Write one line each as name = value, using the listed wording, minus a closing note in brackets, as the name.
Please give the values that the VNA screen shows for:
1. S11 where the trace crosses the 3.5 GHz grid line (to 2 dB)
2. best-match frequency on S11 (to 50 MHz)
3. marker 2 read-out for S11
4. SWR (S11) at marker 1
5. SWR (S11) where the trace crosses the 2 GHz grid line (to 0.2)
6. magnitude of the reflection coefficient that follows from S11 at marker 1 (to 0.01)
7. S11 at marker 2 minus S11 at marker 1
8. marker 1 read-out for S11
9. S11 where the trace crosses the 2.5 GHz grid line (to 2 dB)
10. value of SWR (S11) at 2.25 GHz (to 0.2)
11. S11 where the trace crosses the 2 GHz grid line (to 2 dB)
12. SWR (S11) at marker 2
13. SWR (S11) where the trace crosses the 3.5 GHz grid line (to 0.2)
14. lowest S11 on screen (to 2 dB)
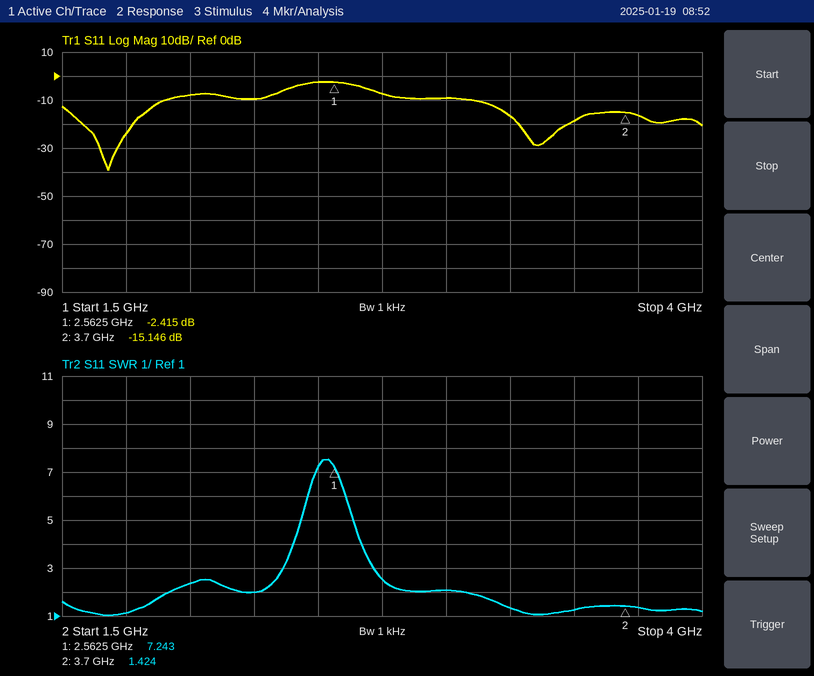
S11 where the trace crosses the 3.5 GHz grid line = -18 dB
best-match frequency on S11 = 1.70 GHz
marker 2 read-out for S11 = -15.146 dB
SWR (S11) at marker 1 = 7.243
SWR (S11) where the trace crosses the 2 GHz grid line = 2.4
magnitude of the reflection coefficient that follows from S11 at marker 1 = 0.76
S11 at marker 2 minus S11 at marker 1 = -12.731 dB
marker 1 read-out for S11 = -2.415 dB
S11 where the trace crosses the 2.5 GHz grid line = -2 dB
value of SWR (S11) at 2.25 GHz = 2.0
S11 where the trace crosses the 2 GHz grid line = -8 dB
SWR (S11) at marker 2 = 1.424
SWR (S11) where the trace crosses the 3.5 GHz grid line = 1.2
lowest S11 on screen = -40 dB
